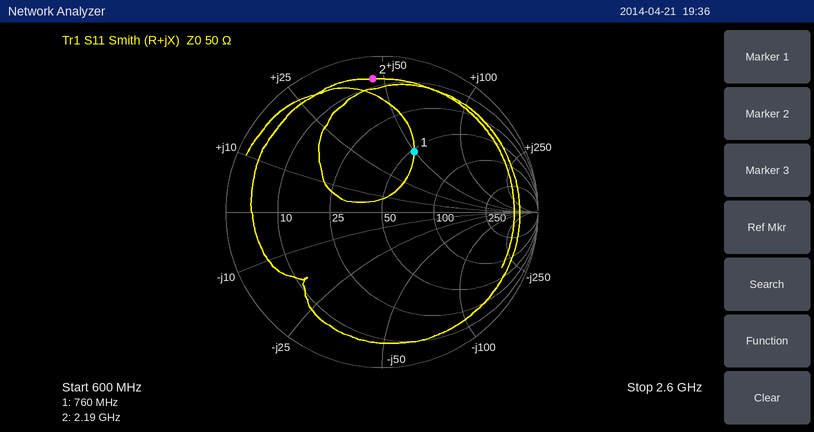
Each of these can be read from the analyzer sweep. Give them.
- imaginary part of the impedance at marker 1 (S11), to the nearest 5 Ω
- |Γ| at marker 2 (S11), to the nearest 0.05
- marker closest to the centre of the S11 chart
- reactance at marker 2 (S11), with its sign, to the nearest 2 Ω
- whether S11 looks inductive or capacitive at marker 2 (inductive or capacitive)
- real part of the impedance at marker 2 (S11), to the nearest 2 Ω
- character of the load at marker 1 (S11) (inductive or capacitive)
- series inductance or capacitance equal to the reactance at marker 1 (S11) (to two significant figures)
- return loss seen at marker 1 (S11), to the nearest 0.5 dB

+50 Ω
0.85
marker 1
+46 Ω
inductive
8 Ω
inductive
10 nH
7.0 dB
